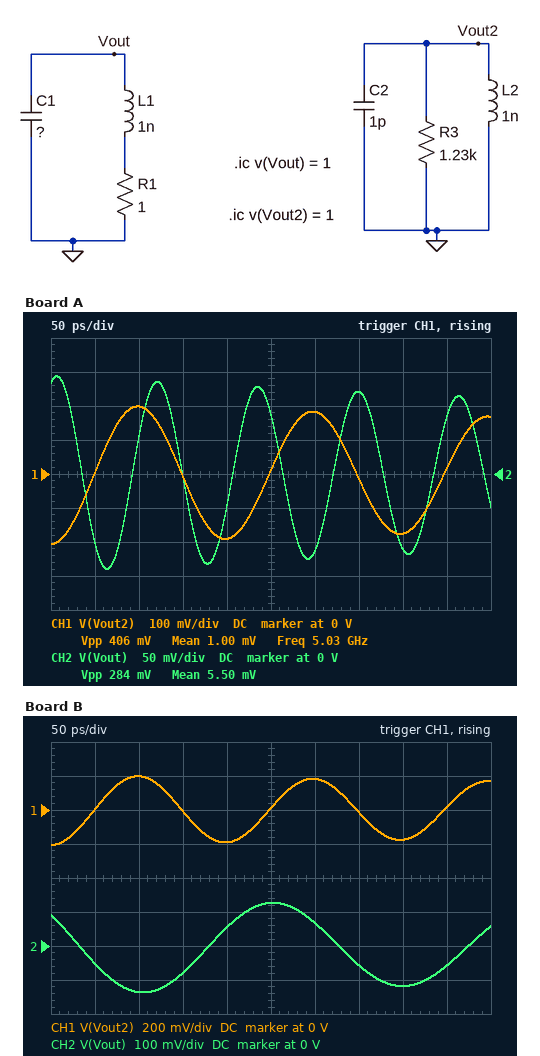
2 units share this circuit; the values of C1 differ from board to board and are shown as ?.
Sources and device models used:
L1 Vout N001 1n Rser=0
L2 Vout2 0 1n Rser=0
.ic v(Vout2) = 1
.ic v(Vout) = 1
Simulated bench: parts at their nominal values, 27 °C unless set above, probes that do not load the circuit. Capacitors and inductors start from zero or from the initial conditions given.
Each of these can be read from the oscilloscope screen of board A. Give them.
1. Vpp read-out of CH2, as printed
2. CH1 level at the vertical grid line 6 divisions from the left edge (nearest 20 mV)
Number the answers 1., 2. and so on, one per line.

1. 284 mV
2. 180 mV
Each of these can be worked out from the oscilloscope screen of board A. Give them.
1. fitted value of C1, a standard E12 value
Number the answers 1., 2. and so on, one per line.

1. 330 fF
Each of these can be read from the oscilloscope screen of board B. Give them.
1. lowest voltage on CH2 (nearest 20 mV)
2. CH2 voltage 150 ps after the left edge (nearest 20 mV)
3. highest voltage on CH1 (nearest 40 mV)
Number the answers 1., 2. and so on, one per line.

1. -140 mV
2. -80 mV
3. 200 mV
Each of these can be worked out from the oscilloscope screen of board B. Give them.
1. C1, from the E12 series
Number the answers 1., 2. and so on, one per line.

1. 2.2 pF
